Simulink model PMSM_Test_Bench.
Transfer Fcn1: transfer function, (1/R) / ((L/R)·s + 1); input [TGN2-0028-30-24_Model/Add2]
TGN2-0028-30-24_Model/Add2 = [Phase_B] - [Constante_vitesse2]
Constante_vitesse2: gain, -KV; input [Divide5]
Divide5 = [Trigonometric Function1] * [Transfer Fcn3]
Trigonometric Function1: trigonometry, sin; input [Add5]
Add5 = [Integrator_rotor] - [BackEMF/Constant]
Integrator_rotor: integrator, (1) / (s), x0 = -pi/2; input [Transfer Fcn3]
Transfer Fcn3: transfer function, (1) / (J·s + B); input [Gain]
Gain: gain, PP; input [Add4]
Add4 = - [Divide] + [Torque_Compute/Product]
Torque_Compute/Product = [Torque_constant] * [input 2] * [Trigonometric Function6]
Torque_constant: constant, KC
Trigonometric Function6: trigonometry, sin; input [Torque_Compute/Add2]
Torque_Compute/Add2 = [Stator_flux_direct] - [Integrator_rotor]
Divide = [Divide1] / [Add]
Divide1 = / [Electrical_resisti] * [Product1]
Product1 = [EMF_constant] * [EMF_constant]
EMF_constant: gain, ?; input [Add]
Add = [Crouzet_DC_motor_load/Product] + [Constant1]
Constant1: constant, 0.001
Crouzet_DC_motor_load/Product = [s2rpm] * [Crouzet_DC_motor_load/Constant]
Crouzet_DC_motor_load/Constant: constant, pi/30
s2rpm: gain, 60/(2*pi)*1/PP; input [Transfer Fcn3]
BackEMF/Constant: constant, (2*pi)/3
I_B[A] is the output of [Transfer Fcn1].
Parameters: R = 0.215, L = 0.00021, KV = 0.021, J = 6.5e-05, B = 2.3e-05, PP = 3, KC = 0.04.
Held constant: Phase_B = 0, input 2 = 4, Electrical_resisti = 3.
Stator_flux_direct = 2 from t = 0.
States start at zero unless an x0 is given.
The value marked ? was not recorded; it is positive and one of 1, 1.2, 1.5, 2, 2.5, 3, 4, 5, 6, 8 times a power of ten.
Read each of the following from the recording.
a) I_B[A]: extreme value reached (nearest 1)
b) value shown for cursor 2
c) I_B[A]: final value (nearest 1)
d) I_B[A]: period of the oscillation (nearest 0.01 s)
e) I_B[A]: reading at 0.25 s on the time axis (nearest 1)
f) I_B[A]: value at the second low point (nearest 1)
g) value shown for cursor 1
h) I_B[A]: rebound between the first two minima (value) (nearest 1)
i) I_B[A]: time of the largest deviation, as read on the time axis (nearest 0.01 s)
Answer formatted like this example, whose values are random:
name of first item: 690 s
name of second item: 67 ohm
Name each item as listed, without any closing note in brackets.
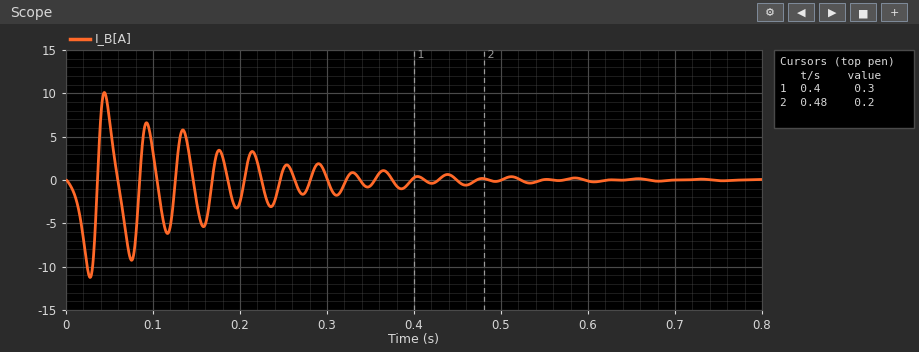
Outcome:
I_B[A]: extreme value reached: -11
value shown for cursor 2: 0.2
I_B[A]: final value: 0
I_B[A]: period of the oscillation: 0.05 s
I_B[A]: reading at 0.25 s on the time axis: 1
I_B[A]: value at the second low point: -9
value shown for cursor 1: 0.3
I_B[A]: rebound between the first two minima (value): 10
I_B[A]: time of the largest deviation, as read on the time axis: 0.03 s
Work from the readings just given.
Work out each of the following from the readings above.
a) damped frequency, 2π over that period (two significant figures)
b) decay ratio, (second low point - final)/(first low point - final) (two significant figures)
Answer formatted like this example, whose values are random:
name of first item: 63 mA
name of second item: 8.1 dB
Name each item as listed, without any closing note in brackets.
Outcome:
damped frequency, 2π over that period: 130 rad/s
decay ratio, (second low point - final)/(first low point - final): 0.82
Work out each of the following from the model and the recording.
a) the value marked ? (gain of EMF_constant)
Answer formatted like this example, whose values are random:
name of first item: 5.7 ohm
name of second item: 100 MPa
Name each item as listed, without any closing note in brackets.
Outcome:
the value marked ?: 0.04
